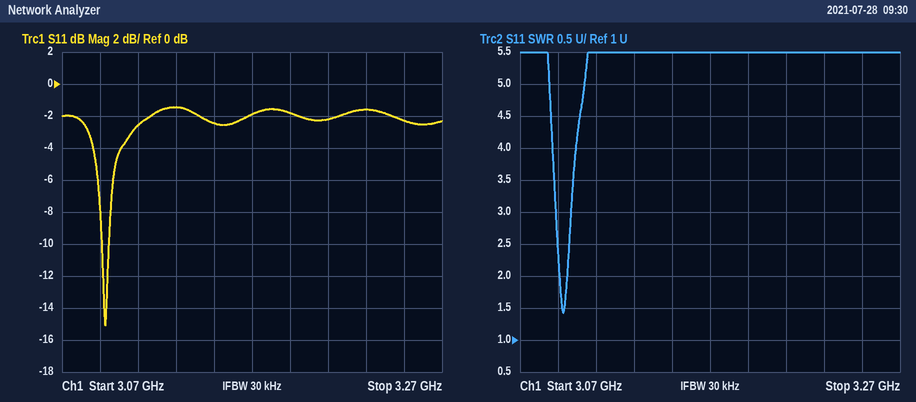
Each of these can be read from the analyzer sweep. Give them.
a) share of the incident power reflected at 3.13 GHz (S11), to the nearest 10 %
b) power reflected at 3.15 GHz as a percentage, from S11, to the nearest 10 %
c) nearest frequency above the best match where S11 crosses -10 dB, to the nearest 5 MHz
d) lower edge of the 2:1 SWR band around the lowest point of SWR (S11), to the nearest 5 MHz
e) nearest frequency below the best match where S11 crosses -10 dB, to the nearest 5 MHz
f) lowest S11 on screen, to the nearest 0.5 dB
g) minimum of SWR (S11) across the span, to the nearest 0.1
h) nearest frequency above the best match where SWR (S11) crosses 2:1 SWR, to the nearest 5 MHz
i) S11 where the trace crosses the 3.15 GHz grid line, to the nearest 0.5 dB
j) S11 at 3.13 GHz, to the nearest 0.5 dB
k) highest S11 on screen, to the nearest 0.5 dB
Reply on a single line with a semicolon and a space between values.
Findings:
70 %; 60 %; 3.095 GHz; 3.090 GHz; 3.090 GHz; -15.0 dB; 1.4; 3.095 GHz; -2.5 dB; -1.5 dB; -1.5 dB
